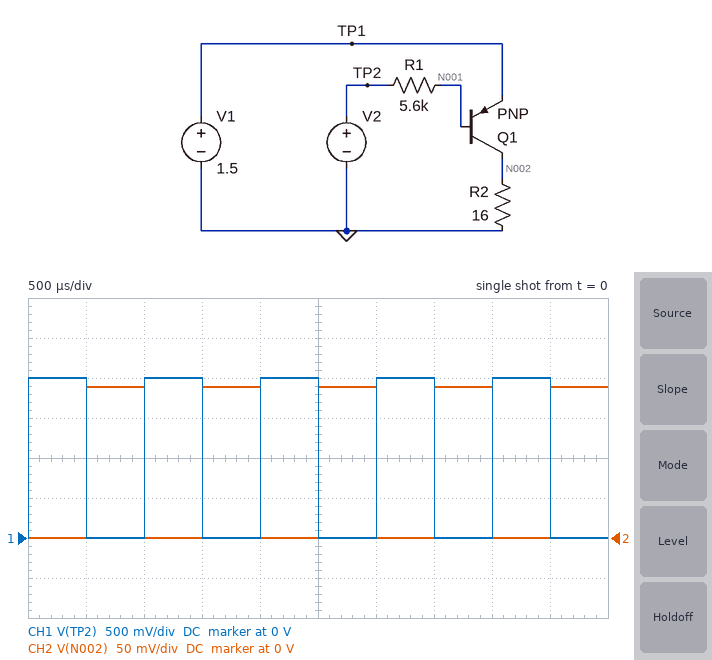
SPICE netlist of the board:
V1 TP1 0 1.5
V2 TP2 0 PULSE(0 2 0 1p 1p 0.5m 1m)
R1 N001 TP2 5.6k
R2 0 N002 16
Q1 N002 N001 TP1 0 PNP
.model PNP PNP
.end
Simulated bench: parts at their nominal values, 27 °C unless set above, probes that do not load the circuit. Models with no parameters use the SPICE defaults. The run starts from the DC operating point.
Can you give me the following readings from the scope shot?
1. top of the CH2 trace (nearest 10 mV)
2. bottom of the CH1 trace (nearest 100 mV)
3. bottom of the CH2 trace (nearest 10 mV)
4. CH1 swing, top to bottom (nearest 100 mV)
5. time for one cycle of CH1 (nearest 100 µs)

190 mV
0 V
0 V
2.0 V
1.0 ms
